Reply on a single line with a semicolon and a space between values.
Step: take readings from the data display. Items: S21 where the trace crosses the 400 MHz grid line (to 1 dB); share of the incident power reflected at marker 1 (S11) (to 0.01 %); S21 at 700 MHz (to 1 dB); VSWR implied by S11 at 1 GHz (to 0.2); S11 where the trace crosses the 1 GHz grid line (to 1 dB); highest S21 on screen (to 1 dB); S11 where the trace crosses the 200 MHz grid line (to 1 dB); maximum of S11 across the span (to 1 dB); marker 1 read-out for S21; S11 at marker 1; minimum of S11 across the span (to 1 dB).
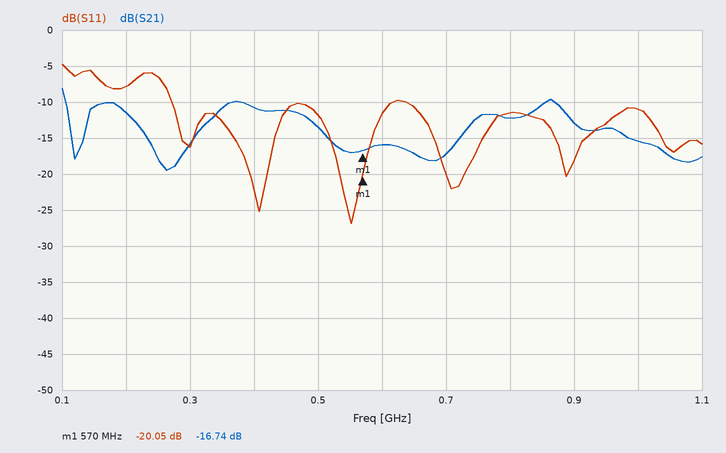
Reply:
-11 dB; 0.99 %; -17 dB; 1.8; -11 dB; -8 dB; -8 dB; -5 dB; -16.74 dB; -20.05 dB; -27 dB
